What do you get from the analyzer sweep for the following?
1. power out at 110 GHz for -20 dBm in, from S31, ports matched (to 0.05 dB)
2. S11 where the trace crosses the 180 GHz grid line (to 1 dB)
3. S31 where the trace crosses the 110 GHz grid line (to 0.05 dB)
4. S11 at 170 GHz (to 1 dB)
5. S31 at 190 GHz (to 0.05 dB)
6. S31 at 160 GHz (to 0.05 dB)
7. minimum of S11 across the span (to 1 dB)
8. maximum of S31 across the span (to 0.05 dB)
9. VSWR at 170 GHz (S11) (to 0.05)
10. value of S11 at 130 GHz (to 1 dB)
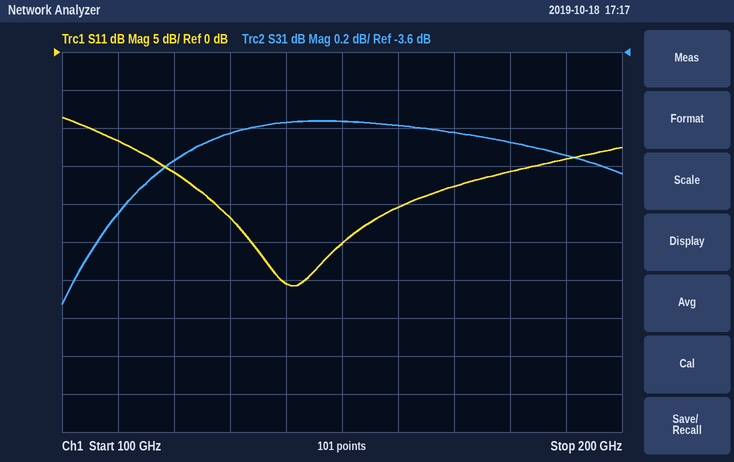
-24.45 dBm
-16 dB
-4.45 dB
-18 dB
-4.15 dB
-4.00 dB
-31 dB
-3.95 dB
1.30
-22 dB
